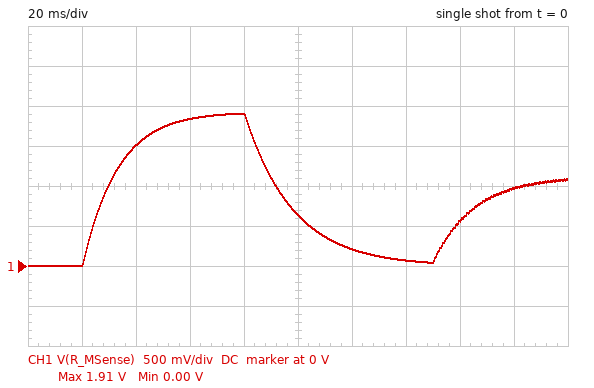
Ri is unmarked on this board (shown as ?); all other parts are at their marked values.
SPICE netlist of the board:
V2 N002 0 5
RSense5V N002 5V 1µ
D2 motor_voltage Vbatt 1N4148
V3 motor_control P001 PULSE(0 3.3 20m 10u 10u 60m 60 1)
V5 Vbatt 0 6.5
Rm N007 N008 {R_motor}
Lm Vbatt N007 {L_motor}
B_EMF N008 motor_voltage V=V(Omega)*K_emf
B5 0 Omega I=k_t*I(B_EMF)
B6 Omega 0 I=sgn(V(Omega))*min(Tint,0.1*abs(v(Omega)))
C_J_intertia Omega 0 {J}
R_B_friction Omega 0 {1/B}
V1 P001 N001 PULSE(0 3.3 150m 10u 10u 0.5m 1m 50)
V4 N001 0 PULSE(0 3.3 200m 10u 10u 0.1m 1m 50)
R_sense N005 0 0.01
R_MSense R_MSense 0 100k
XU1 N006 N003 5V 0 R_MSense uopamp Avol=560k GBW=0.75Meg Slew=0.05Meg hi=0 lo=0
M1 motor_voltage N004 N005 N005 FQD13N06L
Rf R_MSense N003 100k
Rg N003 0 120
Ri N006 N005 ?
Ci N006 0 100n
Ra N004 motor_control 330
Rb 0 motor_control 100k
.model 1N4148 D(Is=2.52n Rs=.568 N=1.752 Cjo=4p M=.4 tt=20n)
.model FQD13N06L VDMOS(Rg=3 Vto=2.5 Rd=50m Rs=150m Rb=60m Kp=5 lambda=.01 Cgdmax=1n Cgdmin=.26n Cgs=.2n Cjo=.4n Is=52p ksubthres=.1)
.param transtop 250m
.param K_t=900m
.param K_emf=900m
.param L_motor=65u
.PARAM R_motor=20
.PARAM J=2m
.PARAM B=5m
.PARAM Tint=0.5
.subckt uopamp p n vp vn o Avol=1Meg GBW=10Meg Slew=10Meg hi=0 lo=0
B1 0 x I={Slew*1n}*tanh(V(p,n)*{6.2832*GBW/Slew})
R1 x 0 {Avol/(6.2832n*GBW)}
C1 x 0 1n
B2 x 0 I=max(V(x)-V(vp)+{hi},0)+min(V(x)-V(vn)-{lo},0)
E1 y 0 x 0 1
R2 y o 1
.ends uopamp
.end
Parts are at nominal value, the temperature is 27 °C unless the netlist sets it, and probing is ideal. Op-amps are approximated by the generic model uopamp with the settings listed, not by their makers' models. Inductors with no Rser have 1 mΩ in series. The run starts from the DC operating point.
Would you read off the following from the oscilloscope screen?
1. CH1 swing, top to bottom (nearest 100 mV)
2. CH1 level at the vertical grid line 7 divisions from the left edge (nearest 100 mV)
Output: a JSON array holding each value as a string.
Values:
["1.9 V", "100 mV"]
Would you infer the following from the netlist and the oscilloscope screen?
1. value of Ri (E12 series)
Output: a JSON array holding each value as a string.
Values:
["180 kΩ"]
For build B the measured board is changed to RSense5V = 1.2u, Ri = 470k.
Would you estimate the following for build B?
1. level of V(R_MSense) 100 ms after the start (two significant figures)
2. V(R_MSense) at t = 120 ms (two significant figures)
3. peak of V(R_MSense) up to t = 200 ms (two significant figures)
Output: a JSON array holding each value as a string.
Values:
["960 mV", "630 mV", "1.5 V"]
